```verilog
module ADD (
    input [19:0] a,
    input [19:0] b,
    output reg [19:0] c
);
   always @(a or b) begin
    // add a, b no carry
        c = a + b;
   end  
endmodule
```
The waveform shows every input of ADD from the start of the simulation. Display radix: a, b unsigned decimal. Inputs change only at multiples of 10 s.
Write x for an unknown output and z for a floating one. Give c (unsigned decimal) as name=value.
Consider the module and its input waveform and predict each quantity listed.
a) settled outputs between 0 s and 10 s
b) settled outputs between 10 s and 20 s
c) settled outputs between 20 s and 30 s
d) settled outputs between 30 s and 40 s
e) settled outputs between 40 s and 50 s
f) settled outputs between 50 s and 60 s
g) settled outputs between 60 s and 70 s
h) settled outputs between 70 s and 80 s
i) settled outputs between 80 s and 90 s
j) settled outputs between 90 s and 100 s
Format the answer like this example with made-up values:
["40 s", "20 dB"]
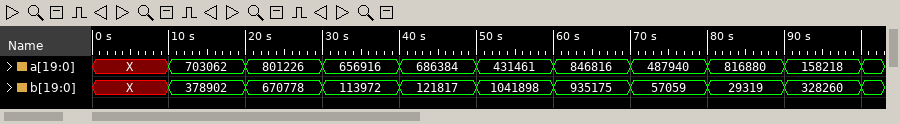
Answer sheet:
["c=x", "c=33388", "c=423428", "c=770888", "c=808201", "c=424783", "c=733415", "c=544999", "c=846199", "c=486478"]
